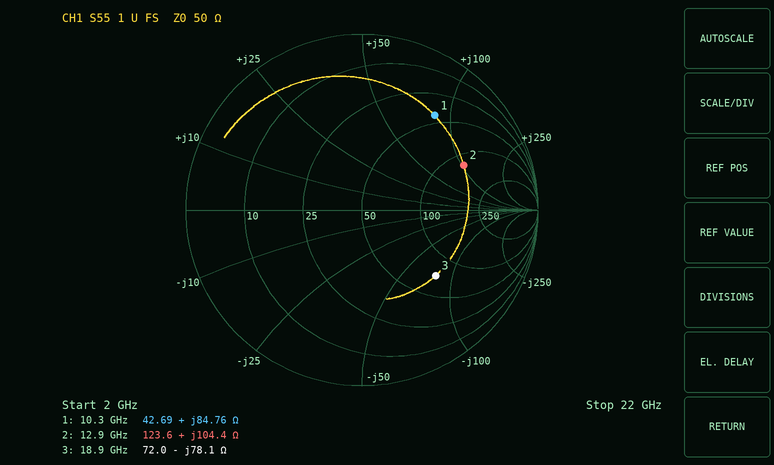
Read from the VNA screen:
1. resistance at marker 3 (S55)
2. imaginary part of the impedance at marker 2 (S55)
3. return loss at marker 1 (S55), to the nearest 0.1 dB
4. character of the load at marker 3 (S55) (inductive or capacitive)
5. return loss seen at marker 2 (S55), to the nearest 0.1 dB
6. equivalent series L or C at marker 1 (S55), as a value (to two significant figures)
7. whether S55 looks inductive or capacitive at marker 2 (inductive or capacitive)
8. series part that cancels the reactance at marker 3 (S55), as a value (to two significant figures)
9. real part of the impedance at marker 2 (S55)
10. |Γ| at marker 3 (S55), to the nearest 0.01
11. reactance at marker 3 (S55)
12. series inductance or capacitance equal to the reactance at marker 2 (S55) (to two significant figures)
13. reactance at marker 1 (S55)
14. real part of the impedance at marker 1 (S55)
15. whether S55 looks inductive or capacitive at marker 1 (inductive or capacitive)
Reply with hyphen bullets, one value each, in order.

- 72.0 Ω
- +104.4 Ω
- 3.4 dB
- capacitive
- 4.0 dB
- 1.3 nH
- inductive
- 660 pH
- 123.6 Ω
- 0.56
- -78.1 Ω
- 1.3 nH
- +84.76 Ω
- 42.69 Ω
- inductive
